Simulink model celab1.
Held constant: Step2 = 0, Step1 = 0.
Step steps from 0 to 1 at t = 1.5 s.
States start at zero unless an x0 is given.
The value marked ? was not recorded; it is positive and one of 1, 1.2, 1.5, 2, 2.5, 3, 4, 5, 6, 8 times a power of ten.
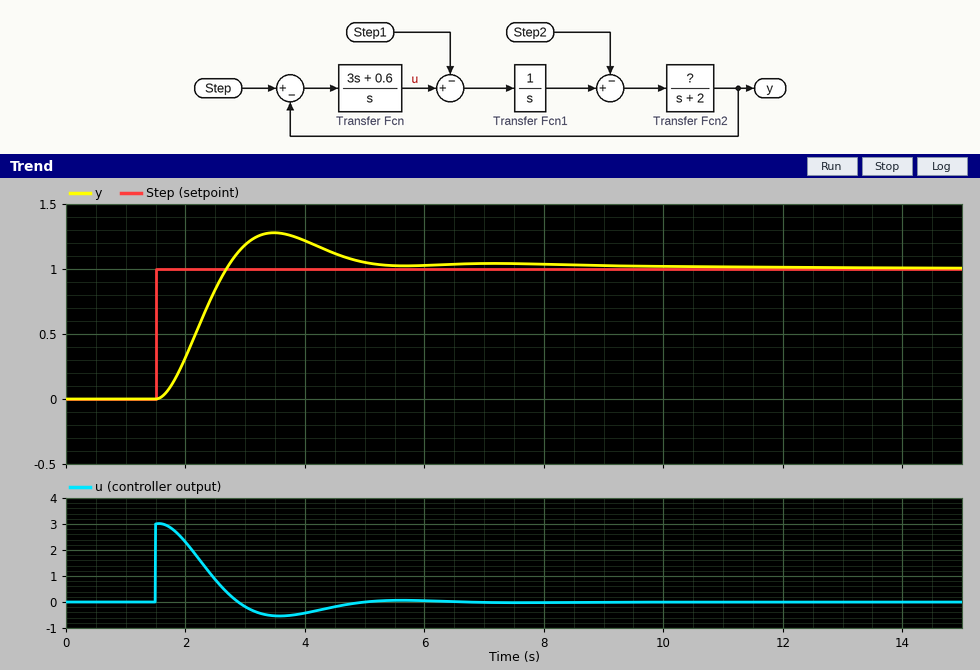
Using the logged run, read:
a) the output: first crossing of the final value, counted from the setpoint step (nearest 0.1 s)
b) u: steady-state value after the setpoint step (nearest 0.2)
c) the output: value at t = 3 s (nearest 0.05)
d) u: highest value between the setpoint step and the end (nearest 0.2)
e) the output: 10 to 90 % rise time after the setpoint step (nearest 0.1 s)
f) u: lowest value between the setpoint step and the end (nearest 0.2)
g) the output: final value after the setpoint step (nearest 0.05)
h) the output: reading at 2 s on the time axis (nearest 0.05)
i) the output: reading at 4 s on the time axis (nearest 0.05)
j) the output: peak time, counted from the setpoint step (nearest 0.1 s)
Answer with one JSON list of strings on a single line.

["1.2 s", "0.0", "1.20", "3.0", "0.8 s", "-0.6", "1.00", "0.30", "1.20", "2.0 s"]
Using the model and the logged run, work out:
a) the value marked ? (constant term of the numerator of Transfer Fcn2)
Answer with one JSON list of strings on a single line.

["1.2"]
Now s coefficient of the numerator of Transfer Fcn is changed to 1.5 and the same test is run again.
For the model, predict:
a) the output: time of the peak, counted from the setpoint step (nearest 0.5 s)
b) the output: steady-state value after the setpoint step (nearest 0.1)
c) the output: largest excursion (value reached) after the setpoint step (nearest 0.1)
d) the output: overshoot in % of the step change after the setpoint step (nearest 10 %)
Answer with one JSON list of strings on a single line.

["3.0 s", "1.0", "1.4", "40 %"]
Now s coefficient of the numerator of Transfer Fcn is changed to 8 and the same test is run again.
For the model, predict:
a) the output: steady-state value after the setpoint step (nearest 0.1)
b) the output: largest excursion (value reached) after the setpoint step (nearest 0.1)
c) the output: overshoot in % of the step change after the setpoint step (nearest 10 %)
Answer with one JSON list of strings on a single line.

["1.0", "1.4", "40 %"]
